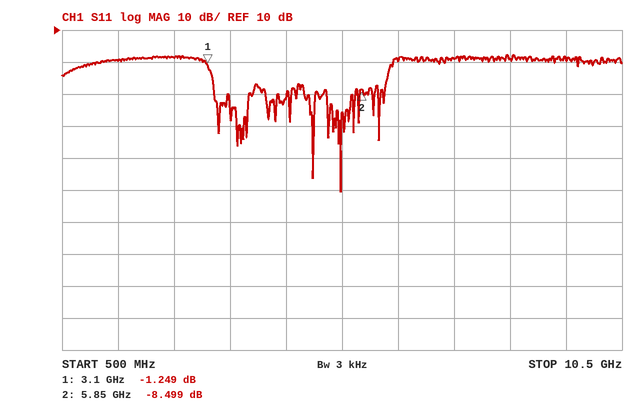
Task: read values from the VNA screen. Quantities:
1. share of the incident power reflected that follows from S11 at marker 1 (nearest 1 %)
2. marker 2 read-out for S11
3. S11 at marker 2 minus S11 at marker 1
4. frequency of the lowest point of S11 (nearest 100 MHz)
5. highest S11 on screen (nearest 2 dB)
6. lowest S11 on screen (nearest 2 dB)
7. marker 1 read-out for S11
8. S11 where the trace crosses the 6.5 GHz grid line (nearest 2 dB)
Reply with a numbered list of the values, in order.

1. 75 %
2. -8.499 dB
3. -7.250 dB
4. 5.5 GHz
5. 2 dB
6. -40 dB
7. -1.249 dB
8. 0 dB
